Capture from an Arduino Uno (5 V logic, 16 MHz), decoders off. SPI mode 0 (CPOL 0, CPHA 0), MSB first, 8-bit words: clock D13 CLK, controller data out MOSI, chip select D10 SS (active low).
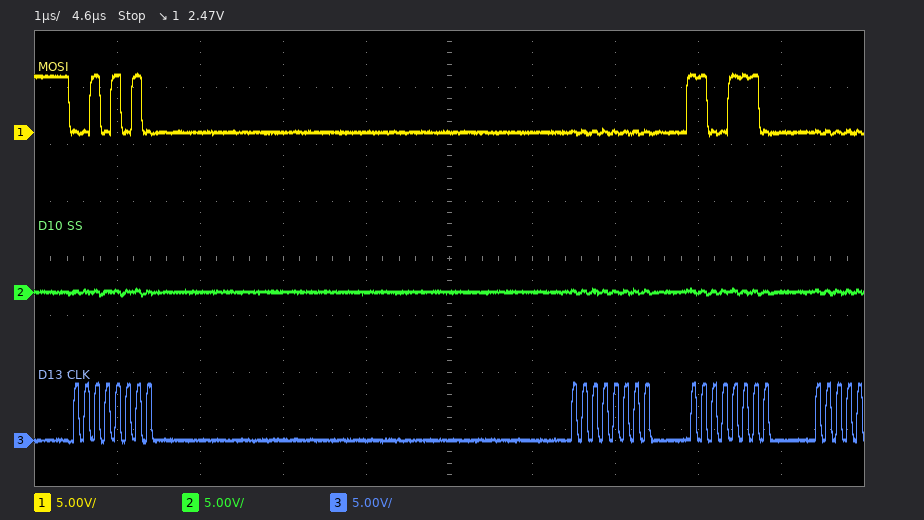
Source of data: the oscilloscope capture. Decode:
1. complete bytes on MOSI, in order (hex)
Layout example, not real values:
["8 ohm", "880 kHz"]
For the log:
["0x2A 0x00 0xCE"]
